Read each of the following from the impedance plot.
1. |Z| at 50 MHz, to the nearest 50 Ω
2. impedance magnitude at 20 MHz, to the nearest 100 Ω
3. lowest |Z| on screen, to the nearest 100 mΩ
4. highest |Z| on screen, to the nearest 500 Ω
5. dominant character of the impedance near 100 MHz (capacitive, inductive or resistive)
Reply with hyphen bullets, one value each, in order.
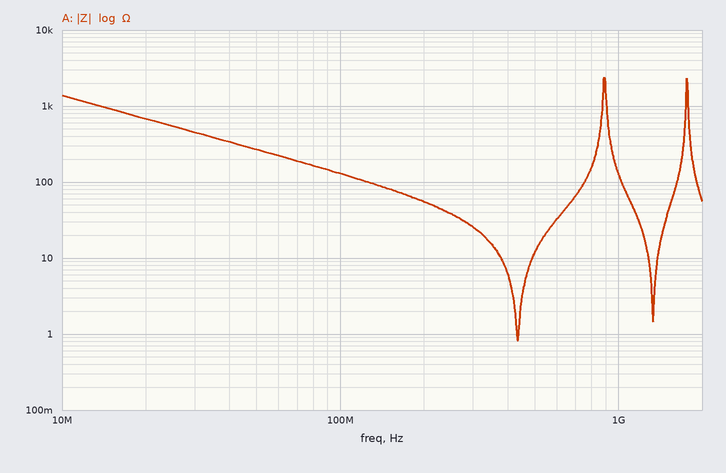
- 250 Ω
- 700 Ω
- 800 mΩ
- 2.5 kΩ
- capacitive
